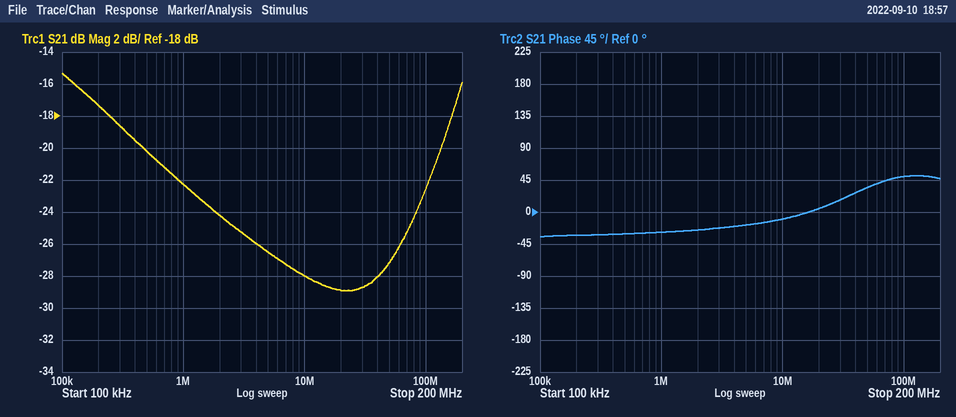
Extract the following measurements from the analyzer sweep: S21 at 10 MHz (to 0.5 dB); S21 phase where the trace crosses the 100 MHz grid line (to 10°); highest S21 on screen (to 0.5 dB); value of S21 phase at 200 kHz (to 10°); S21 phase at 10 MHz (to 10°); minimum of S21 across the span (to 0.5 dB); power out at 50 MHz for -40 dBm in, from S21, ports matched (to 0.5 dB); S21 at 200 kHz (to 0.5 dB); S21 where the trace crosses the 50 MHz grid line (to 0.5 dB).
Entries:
-28.0 dB
50°
-15.5 dB
-30°
-10°
-29.0 dB
-67.0 dBm
-17.5 dB
-27.0 dB
